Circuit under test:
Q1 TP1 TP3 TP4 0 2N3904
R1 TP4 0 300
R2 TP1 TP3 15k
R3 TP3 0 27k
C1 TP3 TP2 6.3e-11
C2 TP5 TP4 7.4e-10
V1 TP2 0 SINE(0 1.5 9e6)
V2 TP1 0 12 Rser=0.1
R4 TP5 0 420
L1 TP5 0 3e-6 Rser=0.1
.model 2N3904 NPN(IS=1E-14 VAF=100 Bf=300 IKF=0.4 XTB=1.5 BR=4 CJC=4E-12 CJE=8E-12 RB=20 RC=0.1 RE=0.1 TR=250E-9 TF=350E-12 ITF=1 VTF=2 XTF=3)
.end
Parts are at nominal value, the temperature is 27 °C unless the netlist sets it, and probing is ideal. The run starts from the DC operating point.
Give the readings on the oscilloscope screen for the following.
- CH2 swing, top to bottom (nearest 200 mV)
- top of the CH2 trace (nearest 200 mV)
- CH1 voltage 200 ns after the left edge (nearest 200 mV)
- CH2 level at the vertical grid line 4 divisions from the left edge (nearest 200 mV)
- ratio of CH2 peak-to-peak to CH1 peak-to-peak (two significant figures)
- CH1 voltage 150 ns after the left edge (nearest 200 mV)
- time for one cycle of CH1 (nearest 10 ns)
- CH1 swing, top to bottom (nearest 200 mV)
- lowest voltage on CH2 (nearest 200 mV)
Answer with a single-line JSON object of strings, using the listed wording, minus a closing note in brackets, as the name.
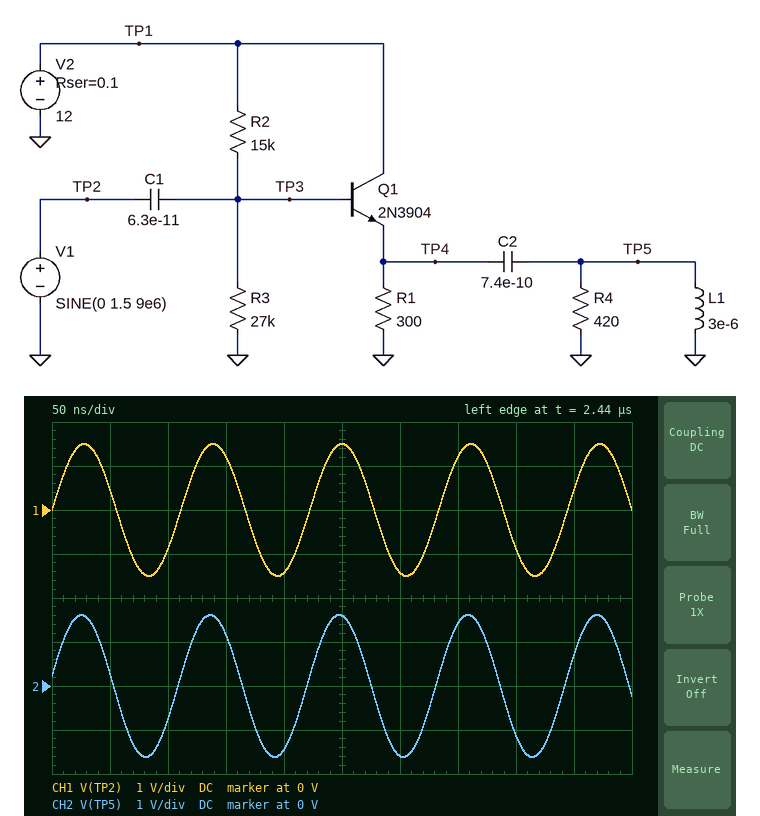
{"CH2 swing, top to bottom": "3.2 V", "top of the CH2 trace": "1.6 V", "CH1 voltage 200 ns after the left edge": "-1.4 V", "CH2 level at the vertical grid line 4 divisions from the left edge": "-1.4 V", "ratio of CH2 peak-to-peak to CH1 peak-to-peak": "1.1", "CH1 voltage 150 ns after the left edge": "1.2 V", "time for one cycle of CH1": "110 ns", "CH1 swing, top to bottom": "3.0 V", "lowest voltage on CH2": "-1.6 V"}
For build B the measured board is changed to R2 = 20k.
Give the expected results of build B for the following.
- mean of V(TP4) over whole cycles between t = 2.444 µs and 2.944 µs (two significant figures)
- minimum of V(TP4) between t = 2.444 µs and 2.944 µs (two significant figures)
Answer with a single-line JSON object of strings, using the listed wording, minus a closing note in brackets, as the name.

{"mean of V(TP4) over whole cycles between t = 2.444 µs and 2.944 µs": "5.5 V", "minimum of V(TP4) between t = 2.444 µs and 2.944 µs": "4.1 V"}
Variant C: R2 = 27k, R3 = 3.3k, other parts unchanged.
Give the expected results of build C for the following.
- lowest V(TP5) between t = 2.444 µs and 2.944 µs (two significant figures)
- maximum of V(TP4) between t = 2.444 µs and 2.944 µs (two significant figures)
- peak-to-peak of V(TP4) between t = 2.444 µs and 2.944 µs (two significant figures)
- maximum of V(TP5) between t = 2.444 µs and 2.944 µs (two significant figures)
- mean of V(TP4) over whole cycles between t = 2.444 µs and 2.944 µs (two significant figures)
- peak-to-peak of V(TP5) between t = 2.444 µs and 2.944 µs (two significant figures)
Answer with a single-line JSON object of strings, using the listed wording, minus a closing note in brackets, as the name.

{"lowest V(TP5) between t = 2.444 µs and 2.944 µs": "-1.1 V", "maximum of V(TP4) between t = 2.444 µs and 2.944 µs": "1.9 V", "peak-to-peak of V(TP4) between t = 2.444 µs and 2.944 µs": "1.8 V", "maximum of V(TP5) between t = 2.444 µs and 2.944 µs": "900 mV", "mean of V(TP4) over whole cycles between t = 2.444 µs and 2.944 µs": "1.1 V", "peak-to-peak of V(TP5) between t = 2.444 µs and 2.944 µs": "2.0 V"}
